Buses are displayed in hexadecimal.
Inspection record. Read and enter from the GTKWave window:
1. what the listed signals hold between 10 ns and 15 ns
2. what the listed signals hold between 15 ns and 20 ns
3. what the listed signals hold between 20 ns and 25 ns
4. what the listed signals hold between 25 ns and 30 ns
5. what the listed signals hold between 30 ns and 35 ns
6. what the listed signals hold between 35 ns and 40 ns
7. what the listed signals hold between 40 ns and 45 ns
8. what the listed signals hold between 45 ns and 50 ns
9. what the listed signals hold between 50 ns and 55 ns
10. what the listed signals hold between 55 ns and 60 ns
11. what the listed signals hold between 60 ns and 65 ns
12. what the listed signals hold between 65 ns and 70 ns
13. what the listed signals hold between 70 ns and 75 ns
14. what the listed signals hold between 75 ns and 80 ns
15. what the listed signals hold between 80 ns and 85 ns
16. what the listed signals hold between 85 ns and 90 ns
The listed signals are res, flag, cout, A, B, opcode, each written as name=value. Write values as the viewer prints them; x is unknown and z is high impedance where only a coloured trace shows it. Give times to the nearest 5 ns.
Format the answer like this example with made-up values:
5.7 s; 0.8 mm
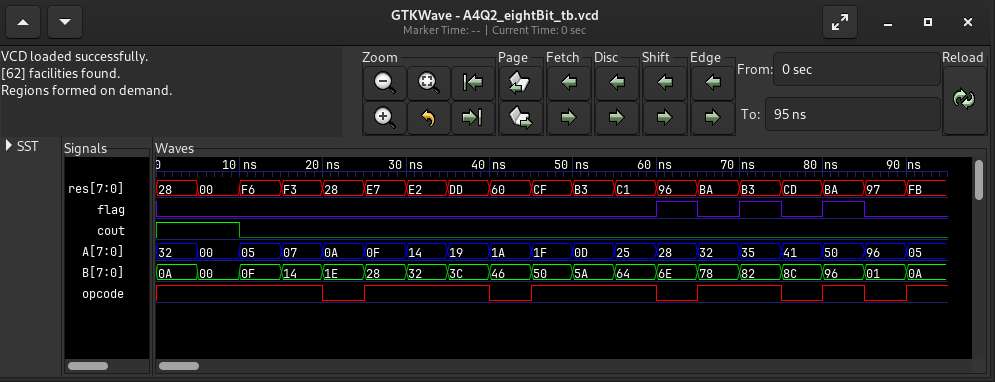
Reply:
res=F6, flag=0, cout=0, A=05, B=0F, opcode=1; res=F3, flag=0, cout=0, A=07, B=14, opcode=1; res=28, flag=0, cout=0, A=0A, B=1E, opcode=0; res=E7, flag=0, cout=0, A=0F, B=28, opcode=1; res=E2, flag=0, cout=0, A=14, B=32, opcode=1; res=DD, flag=0, cout=0, A=19, B=3C, opcode=1; res=60, flag=0, cout=0, A=1A, B=46, opcode=0; res=CF, flag=0, cout=0, A=1F, B=50, opcode=1; res=B3, flag=0, cout=0, A=0D, B=5A, opcode=1; res=C1, flag=0, cout=0, A=25, B=64, opcode=1; res=96, flag=1, cout=0, A=28, B=6E, opcode=0; res=BA, flag=0, cout=0, A=32, B=78, opcode=1; res=B3, flag=1, cout=0, A=35, B=82, opcode=1; res=CD, flag=0, cout=0, A=41, B=8C, opcode=0; res=BA, flag=1, cout=0, A=50, B=96, opcode=1; res=97, flag=0, cout=0, A=96, B=01, opcode=0
